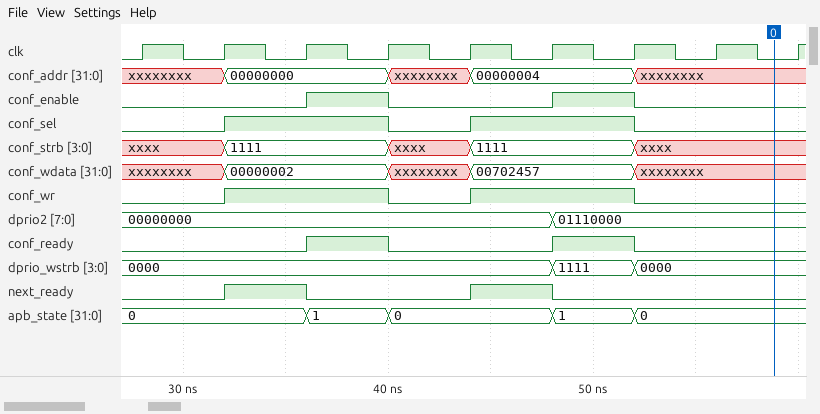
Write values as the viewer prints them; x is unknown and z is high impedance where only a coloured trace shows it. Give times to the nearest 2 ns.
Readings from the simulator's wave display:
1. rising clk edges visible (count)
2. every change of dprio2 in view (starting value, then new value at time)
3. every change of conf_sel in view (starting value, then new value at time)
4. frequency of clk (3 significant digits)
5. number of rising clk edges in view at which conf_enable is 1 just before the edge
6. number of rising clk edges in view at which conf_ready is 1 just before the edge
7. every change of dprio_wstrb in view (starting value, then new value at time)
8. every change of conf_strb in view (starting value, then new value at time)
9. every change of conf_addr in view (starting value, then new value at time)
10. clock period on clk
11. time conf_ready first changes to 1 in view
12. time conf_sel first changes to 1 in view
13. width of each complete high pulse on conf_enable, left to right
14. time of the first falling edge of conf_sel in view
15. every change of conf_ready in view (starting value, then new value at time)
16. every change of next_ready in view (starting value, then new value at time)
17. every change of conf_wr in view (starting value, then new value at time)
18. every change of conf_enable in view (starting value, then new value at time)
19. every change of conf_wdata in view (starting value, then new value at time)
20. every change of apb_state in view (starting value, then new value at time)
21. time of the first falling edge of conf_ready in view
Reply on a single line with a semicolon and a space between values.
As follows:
9; 00000000, 01110000 at 48 ns; 0, 1 at 32 ns, 0 at 40 ns, 1 at 44 ns, 0 at 52 ns; 250 MHz; 2; 2; 0000, 1111 at 48 ns, 0000 at 52 ns; xxxx, 1111 at 32 ns, xxxx at 40 ns, 1111 at 44 ns, xxxx at 52 ns; xxxxxxxx, 00000000 at 32 ns, xxxxxxxx at 40 ns, 00000004 at 44 ns, xxxxxxxx at 52 ns; 4 ns; 36 ns; 32 ns; 4 ns, 4 ns; 40 ns; 0, 1 at 36 ns, 0 at 40 ns, 1 at 48 ns, 0 at 52 ns; 0, 1 at 32 ns, 0 at 36 ns, 1 at 44 ns, 0 at 48 ns; 0, 1 at 32 ns, 0 at 40 ns, 1 at 44 ns, 0 at 52 ns; 0, 1 at 36 ns, 0 at 40 ns, 1 at 48 ns, 0 at 52 ns; xxxxxxxx, 00000002 at 32 ns, xxxxxxxx at 40 ns, 00702457 at 44 ns, xxxxxxxx at 52 ns; 0, 1 at 36 ns, 0 at 40 ns, 1 at 48 ns, 0 at 52 ns; 40 ns
